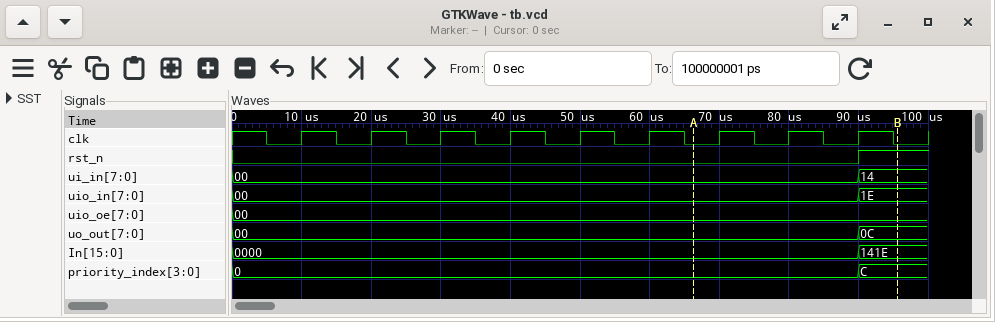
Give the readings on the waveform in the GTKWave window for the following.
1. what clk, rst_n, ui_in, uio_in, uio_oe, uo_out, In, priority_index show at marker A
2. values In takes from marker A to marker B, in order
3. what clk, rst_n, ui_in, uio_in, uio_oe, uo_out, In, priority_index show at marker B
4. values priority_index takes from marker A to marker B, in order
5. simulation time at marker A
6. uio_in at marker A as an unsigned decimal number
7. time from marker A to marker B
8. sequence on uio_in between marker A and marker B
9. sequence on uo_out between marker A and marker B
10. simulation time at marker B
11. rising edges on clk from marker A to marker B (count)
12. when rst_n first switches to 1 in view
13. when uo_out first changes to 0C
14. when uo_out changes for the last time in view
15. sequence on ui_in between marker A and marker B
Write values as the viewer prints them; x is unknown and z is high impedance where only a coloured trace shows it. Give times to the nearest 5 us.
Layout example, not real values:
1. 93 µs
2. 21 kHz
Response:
1. clk=0, rst_n=0, ui_in=00, uio_in=00, uio_oe=00, uo_out=00, In=0000, priority_index=0
2. 0000, 141E
3. clk=0, rst_n=1, ui_in=14, uio_in=1E, uio_oe=00, uo_out=0C, In=141E, priority_index=C
4. 0, C
5. 65 us
6. 0
7. 30 us
8. 00, 1E
9. 00, 0C
10. 95 us
11. 3
12. 90 us
13. 90 us
14. 90 us
15. 00, 14
